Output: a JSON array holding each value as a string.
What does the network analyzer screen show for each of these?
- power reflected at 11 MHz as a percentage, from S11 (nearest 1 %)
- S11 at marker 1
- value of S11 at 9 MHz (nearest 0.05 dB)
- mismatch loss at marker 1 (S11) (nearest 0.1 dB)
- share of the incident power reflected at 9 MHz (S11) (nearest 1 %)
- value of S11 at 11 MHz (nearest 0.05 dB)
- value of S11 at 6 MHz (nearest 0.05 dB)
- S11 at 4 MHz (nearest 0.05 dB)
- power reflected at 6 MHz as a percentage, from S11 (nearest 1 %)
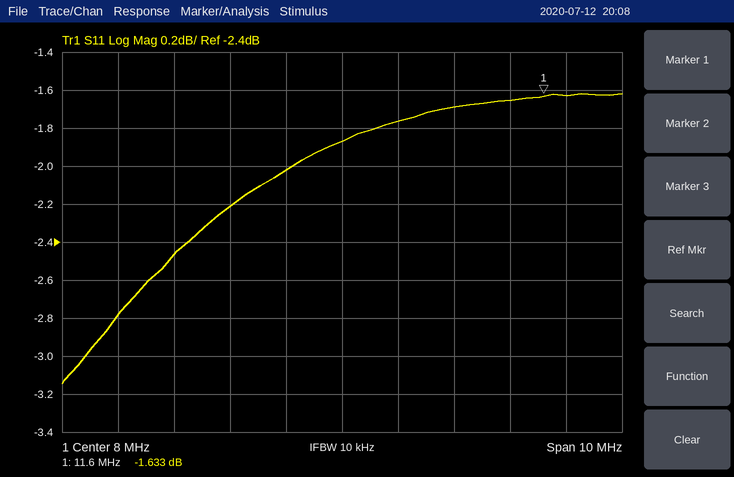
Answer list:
["68 %", "-1.633 dB", "-1.75 dB", "5.0 dB", "67 %", "-1.65 dB", "-2.20 dB", "-2.80 dB", "60 %"]
